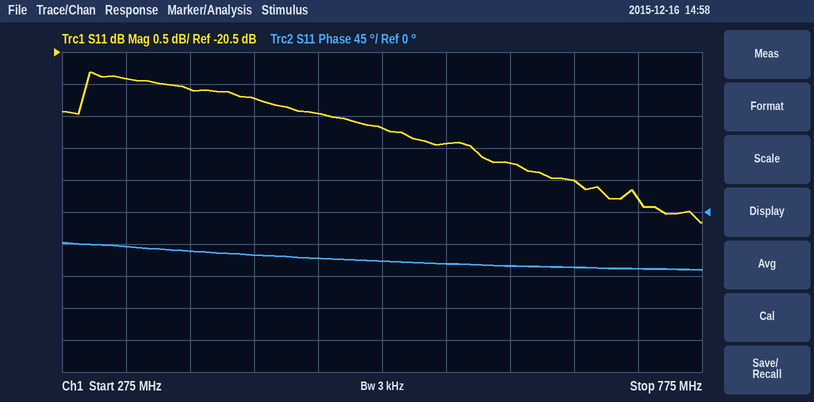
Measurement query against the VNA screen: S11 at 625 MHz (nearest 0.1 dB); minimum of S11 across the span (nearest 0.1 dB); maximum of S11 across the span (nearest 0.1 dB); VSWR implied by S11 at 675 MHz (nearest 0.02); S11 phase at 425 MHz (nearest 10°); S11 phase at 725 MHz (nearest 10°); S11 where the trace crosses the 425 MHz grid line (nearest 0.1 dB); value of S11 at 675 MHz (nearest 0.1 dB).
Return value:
-22.2 dB
-23.2 dB
-20.8 dB
1.16
-60°
-80°
-21.2 dB
-22.5 dB
